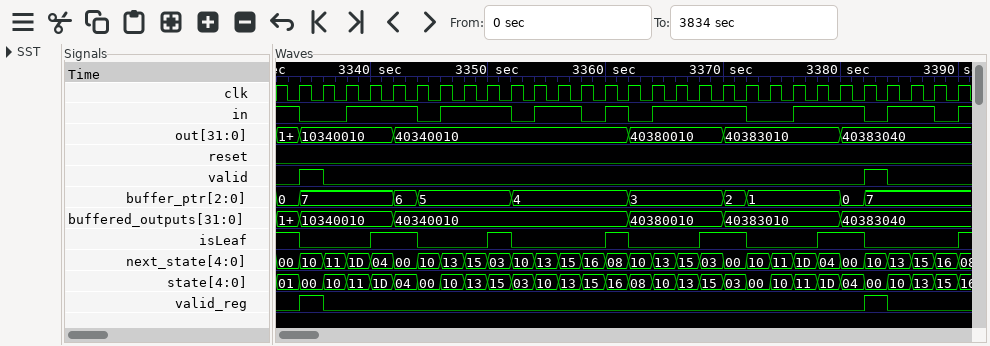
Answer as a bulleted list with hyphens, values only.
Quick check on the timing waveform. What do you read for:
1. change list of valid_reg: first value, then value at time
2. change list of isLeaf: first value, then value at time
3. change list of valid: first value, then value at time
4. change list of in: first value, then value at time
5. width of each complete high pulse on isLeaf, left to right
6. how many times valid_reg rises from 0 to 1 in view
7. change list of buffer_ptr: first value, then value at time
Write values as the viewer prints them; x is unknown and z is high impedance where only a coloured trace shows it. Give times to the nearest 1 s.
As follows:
- 0, 1 at 3334 s, 0 at 3336 s, 1 at 3382 s, 0 at 3384 s
- 1, 0 at 3334 s, 1 at 3340 s, 0 at 3344 s, 1 at 3350 s, 0 at 3352 s, 1 at 3360 s, 0 at 3362 s, 1 at 3368 s, 0 at 3372 s, 1 at 3378 s, 0 at 3382 s, 1 at 3390 s
- 0, 1 at 3334 s, 0 at 3336 s, 1 at 3382 s, 0 at 3384 s
- 1, 0 at 3334 s, 1 at 3338 s, 0 at 3344 s, 1 at 3346 s, 0 at 3352 s, 1 at 3354 s, 0 at 3358 s, 1 at 3360 s, 0 at 3362 s, 1 at 3364 s, 0 at 3372 s, 1 at 3376 s, 0 at 3382 s, 1 at 3384 s, 0 at 3388 s, 1 at 3390 s
- 4 s, 2 s, 2 s, 4 s, 4 s
- 2
- 0, 7 at 3334 s, 6 at 3342 s, 5 at 3344 s, 4 at 3352 s, 3 at 3362 s, 2 at 3370 s, 1 at 3372 s, 0 at 3380 s, 7 at 3382 s
